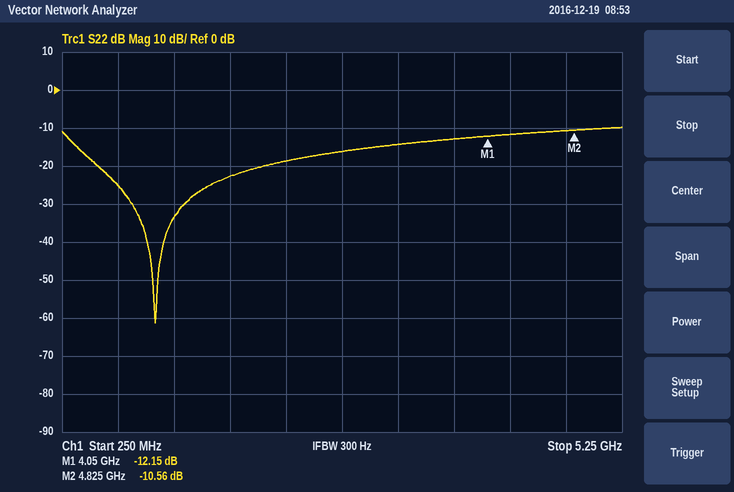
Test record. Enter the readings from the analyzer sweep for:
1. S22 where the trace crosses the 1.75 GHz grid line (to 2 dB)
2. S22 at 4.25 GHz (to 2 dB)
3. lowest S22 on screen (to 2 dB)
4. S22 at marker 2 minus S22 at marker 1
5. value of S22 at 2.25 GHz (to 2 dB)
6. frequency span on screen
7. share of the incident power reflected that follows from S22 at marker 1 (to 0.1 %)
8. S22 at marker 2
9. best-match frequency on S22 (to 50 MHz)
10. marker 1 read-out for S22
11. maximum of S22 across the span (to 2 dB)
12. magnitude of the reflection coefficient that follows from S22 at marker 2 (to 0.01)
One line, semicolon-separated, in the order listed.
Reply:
-22 dB; -12 dB; -62 dB; 1.59 dB; -18 dB; 5 GHz; 6.1 %; -10.56 dB; 1.10 GHz; -12.15 dB; -10 dB; 0.30
